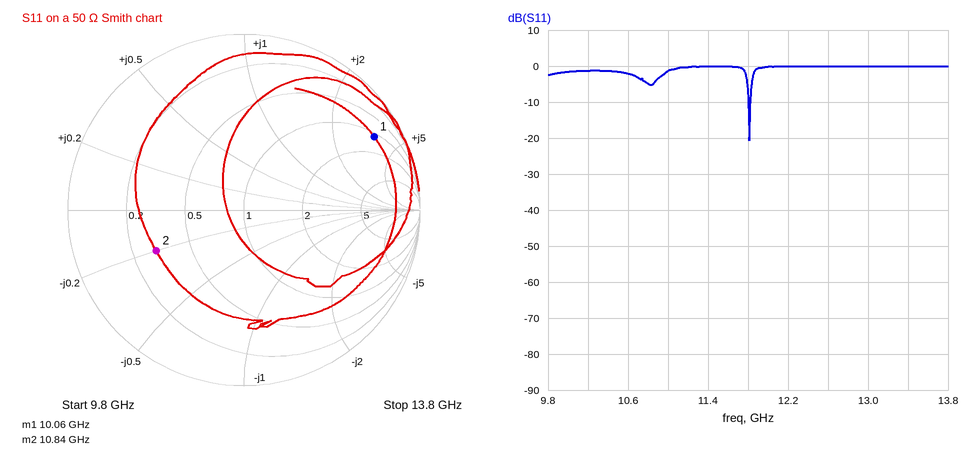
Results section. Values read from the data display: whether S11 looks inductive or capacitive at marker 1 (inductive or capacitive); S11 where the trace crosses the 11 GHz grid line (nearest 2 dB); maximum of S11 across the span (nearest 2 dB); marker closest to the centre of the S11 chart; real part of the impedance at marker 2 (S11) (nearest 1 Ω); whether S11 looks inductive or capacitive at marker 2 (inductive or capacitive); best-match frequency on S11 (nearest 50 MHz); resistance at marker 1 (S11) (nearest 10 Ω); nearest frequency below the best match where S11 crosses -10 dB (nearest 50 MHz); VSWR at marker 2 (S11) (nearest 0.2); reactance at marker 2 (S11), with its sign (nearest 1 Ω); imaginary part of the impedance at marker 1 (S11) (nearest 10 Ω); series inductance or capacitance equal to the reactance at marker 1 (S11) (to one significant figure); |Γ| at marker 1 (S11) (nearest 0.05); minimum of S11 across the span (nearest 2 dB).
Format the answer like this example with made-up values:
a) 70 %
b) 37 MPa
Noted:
a) inductive
b) -2 dB
c) 0 dB
d) marker 2
e) 15 Ω
f) capacitive
g) 11.80 GHz
h) 60 Ω
i) 11.80 GHz
j) 3.4
k) -10 Ω
l) +170 Ω
m) 3 nH
n) 0.85
o) -20 dB
